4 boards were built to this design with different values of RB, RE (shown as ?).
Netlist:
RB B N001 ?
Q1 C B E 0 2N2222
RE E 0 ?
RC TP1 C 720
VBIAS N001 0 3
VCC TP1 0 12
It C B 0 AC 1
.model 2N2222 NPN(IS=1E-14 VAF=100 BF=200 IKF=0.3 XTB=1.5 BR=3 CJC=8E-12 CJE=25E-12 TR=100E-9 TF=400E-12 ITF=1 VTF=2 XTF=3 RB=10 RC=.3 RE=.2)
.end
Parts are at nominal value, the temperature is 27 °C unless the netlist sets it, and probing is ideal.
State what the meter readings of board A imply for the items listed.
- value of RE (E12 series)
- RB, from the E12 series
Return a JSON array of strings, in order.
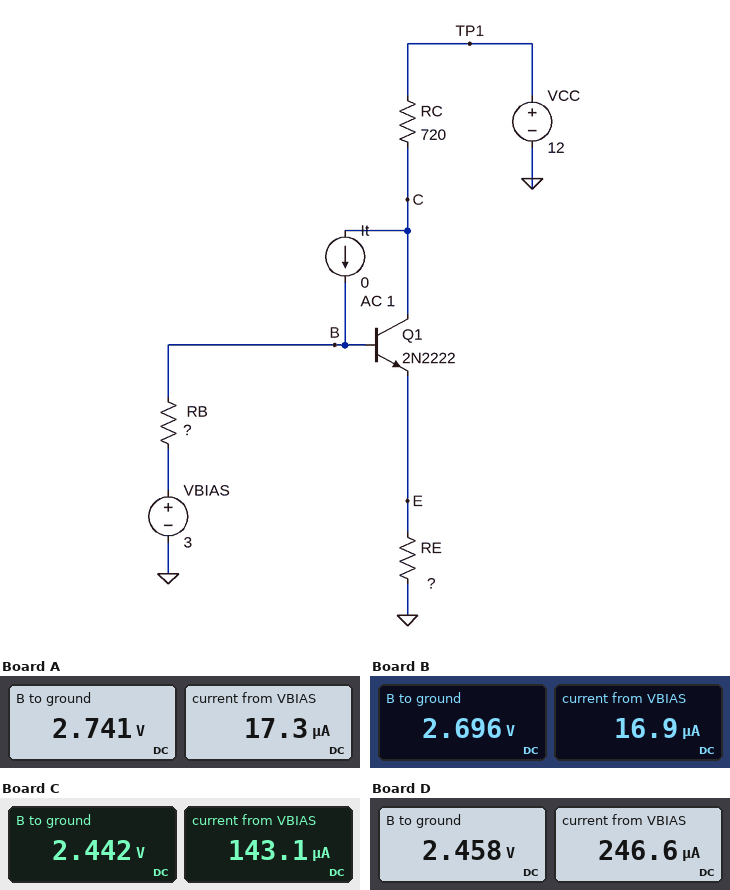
["560 Ω", "15 kΩ"]
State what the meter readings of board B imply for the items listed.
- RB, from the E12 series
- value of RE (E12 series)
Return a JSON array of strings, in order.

["18 kΩ", "560 Ω"]
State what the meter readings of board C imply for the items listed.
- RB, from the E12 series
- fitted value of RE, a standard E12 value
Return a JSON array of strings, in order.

["3.9 kΩ", "120 Ω"]
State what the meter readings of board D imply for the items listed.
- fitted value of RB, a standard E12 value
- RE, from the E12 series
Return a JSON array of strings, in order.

["2.2 kΩ", "120 Ω"]
